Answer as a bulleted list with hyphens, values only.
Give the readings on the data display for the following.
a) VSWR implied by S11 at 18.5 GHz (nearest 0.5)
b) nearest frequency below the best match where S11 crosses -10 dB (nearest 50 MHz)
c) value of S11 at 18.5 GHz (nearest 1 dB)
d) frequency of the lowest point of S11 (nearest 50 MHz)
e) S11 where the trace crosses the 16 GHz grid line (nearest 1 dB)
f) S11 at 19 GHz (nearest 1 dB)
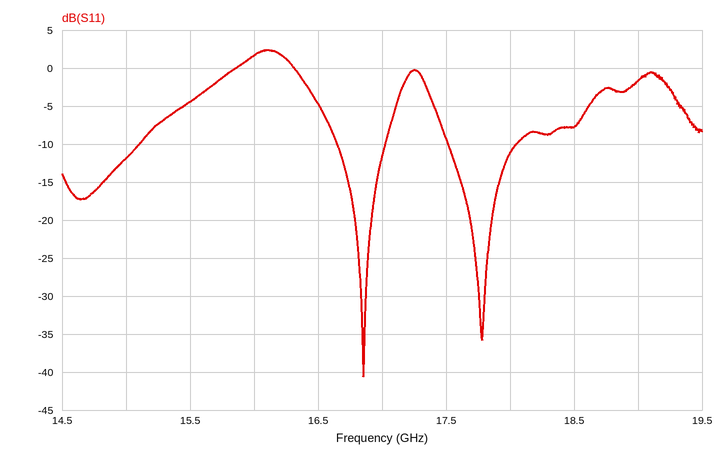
- 2.5
- 16.65 GHz
- -8 dB
- 16.85 GHz
- 2 dB
- -2 dB
